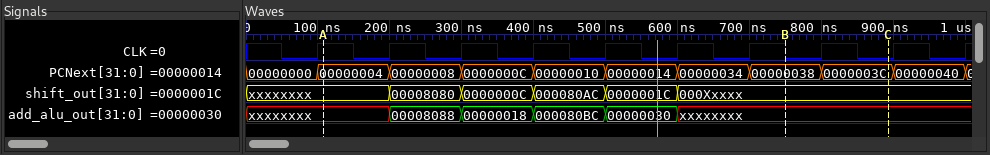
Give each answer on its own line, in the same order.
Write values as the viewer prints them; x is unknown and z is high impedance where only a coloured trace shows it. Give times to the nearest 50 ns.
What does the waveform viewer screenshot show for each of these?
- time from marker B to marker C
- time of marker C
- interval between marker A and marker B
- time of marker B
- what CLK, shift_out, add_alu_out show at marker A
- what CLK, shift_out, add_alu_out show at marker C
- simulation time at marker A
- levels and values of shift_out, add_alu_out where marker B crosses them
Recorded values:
150 ns
900 ns
650 ns
750 ns
CLK=1, shift_out=xxxxxxxx, add_alu_out=xxxxxxxx
CLK=0, shift_out=000Xxxxx, add_alu_out=xxxxxxxx
100 ns
shift_out=000Xxxxx, add_alu_out=xxxxxxxx
